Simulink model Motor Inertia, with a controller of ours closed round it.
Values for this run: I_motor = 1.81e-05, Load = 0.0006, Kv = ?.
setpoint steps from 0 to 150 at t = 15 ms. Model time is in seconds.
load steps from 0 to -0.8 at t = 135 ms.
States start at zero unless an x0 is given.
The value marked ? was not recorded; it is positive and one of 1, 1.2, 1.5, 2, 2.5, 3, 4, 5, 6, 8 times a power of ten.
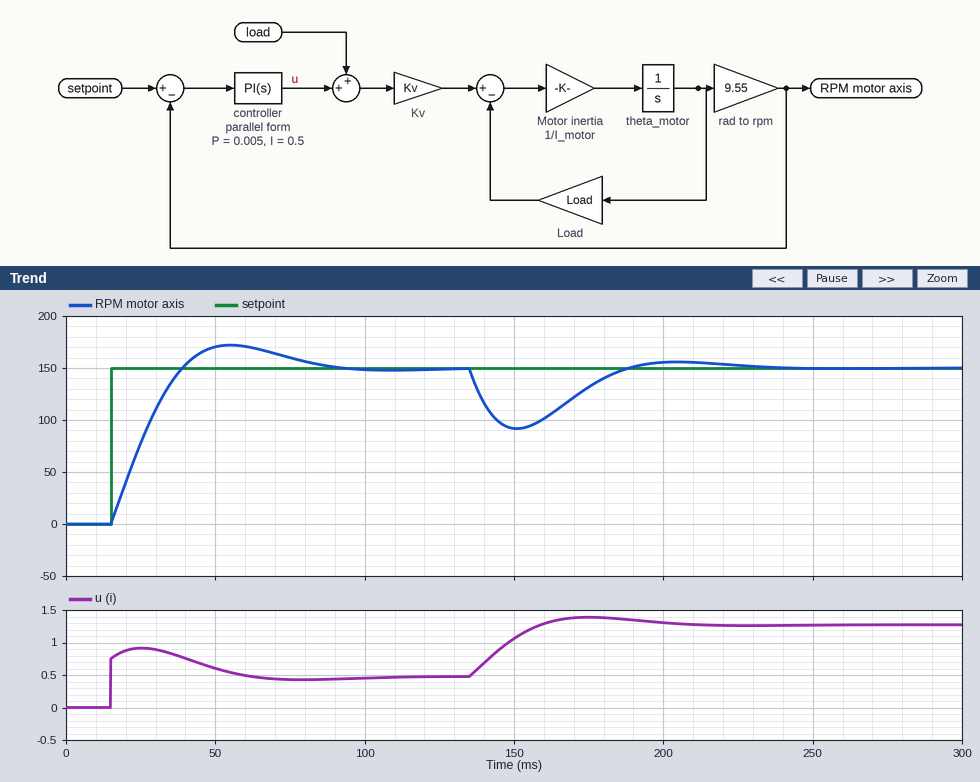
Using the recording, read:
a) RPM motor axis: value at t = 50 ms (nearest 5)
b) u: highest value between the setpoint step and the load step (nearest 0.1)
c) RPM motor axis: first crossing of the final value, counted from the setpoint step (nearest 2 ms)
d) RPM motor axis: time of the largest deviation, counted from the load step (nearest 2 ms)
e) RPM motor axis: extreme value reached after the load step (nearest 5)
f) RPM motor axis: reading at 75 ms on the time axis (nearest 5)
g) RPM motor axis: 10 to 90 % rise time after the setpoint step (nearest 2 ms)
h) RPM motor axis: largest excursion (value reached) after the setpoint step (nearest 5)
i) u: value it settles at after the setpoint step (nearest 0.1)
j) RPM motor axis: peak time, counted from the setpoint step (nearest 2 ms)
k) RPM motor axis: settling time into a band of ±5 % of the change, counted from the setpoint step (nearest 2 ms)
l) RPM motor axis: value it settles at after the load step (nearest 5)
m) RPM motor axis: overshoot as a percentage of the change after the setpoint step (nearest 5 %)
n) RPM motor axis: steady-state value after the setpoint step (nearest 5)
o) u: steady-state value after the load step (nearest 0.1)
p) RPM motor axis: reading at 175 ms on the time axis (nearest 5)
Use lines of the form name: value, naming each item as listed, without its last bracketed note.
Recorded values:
RPM motor axis: value at t = 50 ms: 170
u: highest value between the setpoint step and the load step: 0.9
RPM motor axis: first crossing of the final value, counted from the setpoint step: 24 ms
RPM motor axis: time of the largest deviation, counted from the load step: 16 ms
RPM motor axis: extreme value reached after the load step: 90
RPM motor axis: reading at 75 ms on the time axis: 160
RPM motor axis: 10 to 90 % rise time after the setpoint step: 18 ms
RPM motor axis: largest excursion (value reached) after the setpoint step: 170
u: value it settles at after the setpoint step: 0.5
RPM motor axis: peak time, counted from the setpoint step: 40 ms
RPM motor axis: settling time into a band of ±5 % of the change, counted from the setpoint step: 64 ms
RPM motor axis: value it settles at after the load step: 150
RPM motor axis: overshoot as a percentage of the change after the setpoint step: 15 %
RPM motor axis: steady-state value after the setpoint step: 150
u: steady-state value after the load step: 1.3
RPM motor axis: reading at 175 ms on the time axis: 130
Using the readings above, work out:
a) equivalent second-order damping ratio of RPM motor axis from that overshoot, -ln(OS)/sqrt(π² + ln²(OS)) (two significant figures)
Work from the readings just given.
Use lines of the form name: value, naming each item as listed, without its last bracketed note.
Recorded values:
equivalent second-order damping ratio of RPM motor axis from that overshoot, -ln(OS)/sqrt(π² + ln²(OS)): 0.52
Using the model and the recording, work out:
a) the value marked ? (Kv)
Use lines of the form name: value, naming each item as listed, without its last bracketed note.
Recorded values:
the value marked ?: 0.02
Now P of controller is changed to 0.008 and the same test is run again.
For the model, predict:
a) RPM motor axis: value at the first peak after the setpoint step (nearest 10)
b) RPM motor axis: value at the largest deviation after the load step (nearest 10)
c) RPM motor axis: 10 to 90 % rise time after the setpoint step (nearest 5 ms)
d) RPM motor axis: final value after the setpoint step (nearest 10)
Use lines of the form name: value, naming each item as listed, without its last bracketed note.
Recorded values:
RPM motor axis: value at the first peak after the setpoint step: 160
RPM motor axis: value at the largest deviation after the load step: 100
RPM motor axis: 10 to 90 % rise time after the setpoint step: 15 ms
RPM motor axis: final value after the setpoint step: 150
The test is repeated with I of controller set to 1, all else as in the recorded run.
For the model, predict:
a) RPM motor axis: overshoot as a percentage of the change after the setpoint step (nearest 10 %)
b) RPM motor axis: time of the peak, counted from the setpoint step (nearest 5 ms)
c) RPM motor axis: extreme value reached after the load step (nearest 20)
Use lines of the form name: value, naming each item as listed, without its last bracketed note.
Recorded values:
RPM motor axis: overshoot as a percentage of the change after the setpoint step: 30 %
RPM motor axis: time of the peak, counted from the setpoint step: 30 ms
RPM motor axis: extreme value reached after the load step: 100
